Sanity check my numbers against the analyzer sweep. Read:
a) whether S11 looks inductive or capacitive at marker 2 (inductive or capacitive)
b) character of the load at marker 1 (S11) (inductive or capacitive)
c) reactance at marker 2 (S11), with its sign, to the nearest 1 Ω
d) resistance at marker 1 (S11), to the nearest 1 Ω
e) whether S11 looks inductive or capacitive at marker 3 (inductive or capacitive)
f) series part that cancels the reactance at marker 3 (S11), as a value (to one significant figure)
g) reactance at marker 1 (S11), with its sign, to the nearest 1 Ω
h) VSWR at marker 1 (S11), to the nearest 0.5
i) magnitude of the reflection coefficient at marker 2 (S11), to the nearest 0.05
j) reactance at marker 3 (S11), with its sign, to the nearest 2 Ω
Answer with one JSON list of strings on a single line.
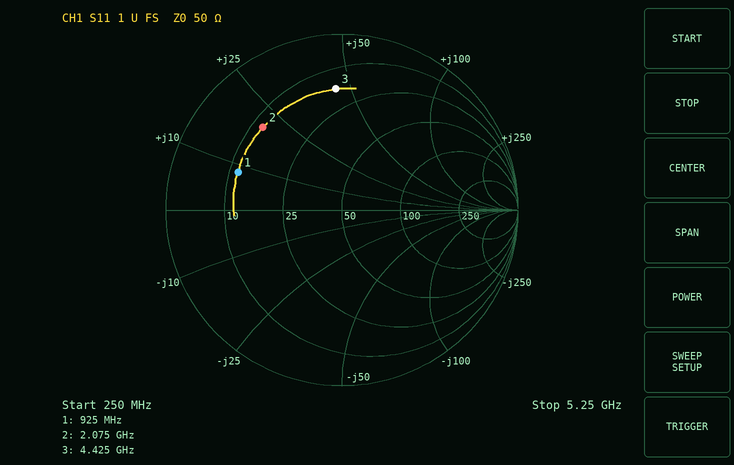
["inductive", "inductive", "+20 Ω", "12 Ω", "inductive", "800 fF", "+8 Ω", "4.5", "0.65", "+44 Ω"]
